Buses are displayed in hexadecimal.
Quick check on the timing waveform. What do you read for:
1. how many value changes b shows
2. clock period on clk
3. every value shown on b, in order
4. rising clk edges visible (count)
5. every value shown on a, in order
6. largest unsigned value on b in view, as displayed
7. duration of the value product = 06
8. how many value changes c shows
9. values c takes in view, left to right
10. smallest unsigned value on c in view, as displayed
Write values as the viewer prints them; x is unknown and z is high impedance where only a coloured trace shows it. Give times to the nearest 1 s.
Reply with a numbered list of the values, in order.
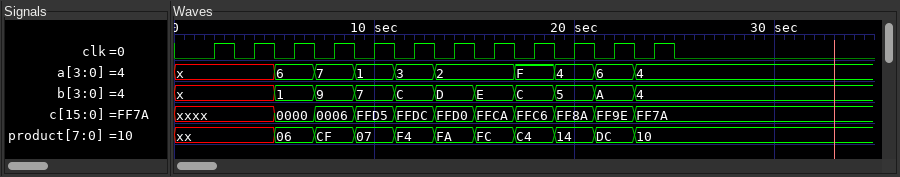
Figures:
1. 10
2. 2 s
3. x, 1, 9, 7, C, D, E, C, 5, A, 4
4. 12
5. x, 6, 7, 1, 3, 2, F, 4, 6, 4
6. E
7. 2 s
8. 10
9. xxxx, 0000, 0006, FFD5, FFDC, FFD0, FFCA, FFC6, FF8A, FF9E, FF7A
10. 0000
